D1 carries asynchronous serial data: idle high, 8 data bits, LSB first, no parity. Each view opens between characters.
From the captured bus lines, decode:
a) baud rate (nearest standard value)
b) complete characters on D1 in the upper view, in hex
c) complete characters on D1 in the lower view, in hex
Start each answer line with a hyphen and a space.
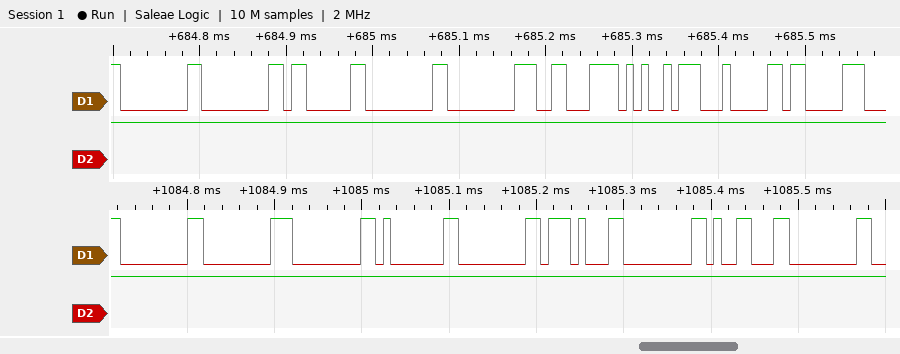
- 115200 baud
- 00, 00, 03, 00, 00, C6, A5, 04, 83
- 00, 00, 00, 01, 00, 17, 00, 19, 00
